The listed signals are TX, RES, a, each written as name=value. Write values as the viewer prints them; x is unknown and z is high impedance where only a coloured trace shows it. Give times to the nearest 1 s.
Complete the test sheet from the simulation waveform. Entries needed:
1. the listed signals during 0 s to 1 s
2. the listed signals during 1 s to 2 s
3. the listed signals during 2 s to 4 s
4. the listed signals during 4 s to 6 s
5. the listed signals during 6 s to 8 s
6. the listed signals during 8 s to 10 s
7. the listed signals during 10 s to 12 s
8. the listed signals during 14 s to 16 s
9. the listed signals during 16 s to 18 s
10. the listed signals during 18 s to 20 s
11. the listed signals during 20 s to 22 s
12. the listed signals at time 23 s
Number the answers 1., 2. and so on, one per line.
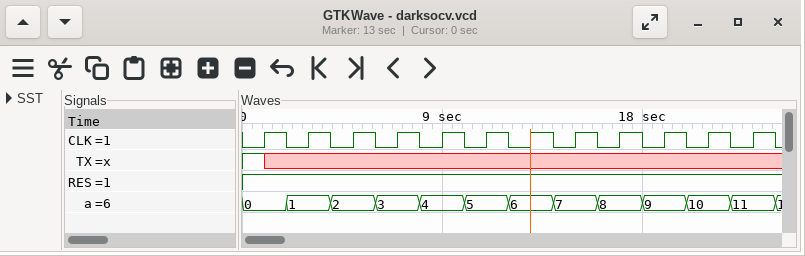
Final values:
1. TX=1, RES=1, a=0
2. TX=x, RES=1, a=0
3. TX=x, RES=1, a=1
4. TX=x, RES=1, a=2
5. TX=x, RES=1, a=3
6. TX=x, RES=1, a=4
7. TX=x, RES=1, a=5
8. TX=x, RES=1, a=7
9. TX=x, RES=1, a=8
10. TX=x, RES=1, a=9
11. TX=x, RES=1, a=10
12. TX=x, RES=1, a=11
